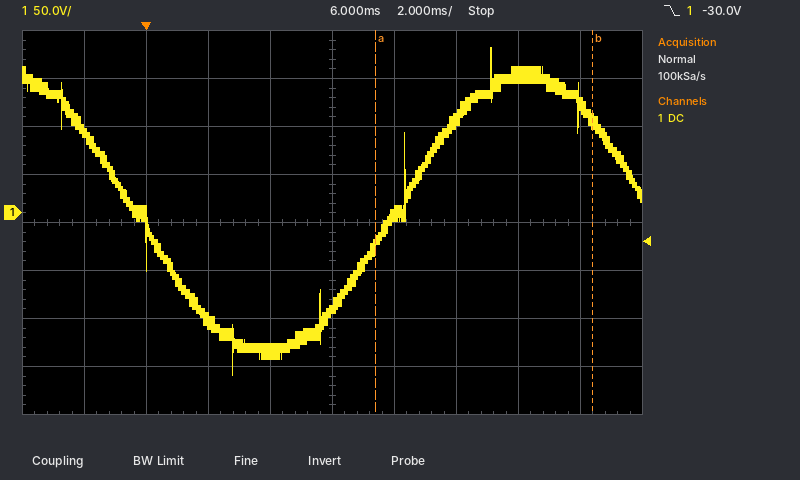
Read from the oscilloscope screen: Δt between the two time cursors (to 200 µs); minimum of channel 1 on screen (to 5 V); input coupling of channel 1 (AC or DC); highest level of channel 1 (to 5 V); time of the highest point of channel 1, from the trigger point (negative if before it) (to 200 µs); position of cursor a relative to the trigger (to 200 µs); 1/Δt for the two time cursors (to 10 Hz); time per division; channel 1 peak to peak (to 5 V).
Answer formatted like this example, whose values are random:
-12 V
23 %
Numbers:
7.0 ms
-170 V
DC
170 V
+11.2 ms
+7.4 ms
140 Hz
2 ms
340 V
